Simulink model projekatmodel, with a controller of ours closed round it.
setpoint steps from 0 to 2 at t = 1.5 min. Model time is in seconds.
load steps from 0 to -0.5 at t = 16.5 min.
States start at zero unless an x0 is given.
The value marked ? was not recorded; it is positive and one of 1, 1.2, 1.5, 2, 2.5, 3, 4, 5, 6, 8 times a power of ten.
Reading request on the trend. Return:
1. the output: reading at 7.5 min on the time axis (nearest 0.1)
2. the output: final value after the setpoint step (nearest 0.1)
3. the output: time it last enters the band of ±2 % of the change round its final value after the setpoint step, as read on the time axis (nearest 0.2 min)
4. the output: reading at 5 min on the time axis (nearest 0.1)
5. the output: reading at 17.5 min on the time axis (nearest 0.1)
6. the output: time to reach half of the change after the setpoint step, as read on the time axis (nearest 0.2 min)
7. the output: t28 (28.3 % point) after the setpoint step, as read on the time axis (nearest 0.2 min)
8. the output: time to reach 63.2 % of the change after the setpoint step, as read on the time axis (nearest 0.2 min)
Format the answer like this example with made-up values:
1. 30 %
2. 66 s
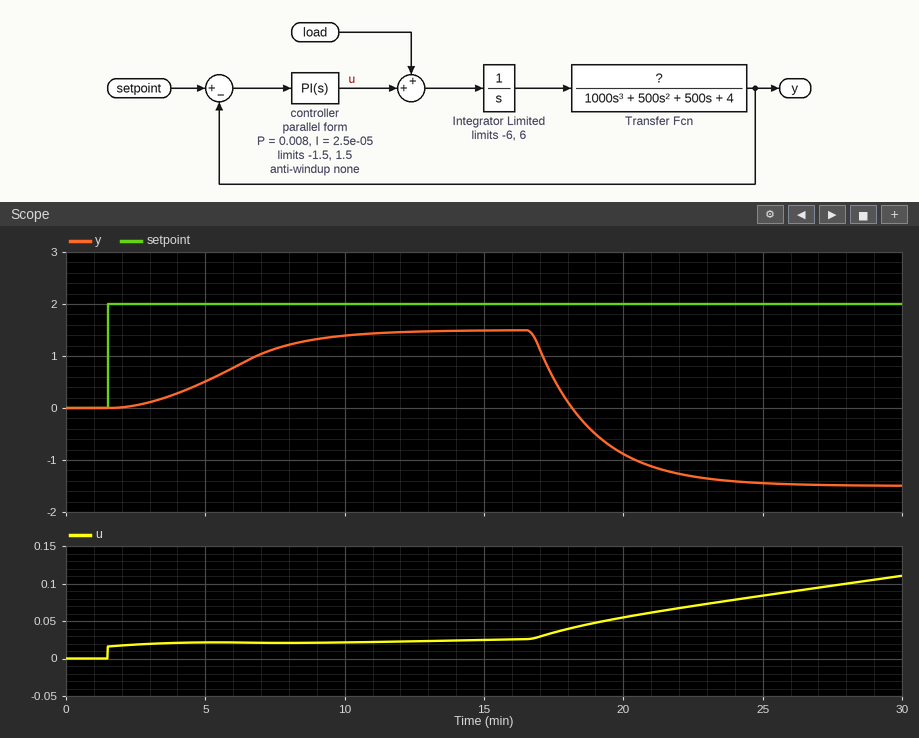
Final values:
1. 1.1
2. 1.5
3. 12.6 min
4. 0.5
5. 0.6
6. 6.0 min
7. 4.6 min
8. 6.6 min
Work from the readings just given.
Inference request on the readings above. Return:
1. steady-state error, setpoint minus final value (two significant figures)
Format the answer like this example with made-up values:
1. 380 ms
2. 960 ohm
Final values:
1. 0.50
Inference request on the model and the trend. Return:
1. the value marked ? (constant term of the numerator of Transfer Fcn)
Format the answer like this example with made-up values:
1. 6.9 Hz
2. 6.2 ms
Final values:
1. 1
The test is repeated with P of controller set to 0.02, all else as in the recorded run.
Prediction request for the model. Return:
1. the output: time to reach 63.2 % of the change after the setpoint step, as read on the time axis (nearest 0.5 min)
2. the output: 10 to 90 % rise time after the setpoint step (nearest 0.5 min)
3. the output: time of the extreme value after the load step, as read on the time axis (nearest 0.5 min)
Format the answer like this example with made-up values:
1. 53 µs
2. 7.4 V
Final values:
1. 5.0 min
2. 5.0 min
3. 30.0 min
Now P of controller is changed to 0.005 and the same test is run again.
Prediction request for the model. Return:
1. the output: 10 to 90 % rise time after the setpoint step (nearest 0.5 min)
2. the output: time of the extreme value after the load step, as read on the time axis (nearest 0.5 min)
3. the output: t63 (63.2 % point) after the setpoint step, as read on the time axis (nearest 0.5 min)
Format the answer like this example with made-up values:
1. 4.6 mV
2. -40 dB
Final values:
1. 6.5 min
2. 30.0 min
3. 7.5 min
